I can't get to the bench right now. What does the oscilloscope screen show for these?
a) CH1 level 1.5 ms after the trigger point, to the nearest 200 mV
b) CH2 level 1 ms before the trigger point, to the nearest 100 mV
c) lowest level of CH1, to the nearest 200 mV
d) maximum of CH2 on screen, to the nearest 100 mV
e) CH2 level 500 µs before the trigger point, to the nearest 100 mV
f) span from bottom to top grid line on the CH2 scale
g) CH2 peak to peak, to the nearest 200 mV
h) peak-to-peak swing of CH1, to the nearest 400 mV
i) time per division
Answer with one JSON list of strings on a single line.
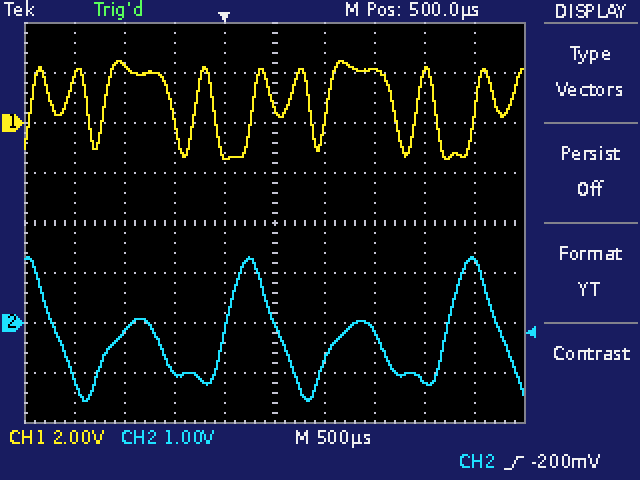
["2.2 V", "-200 mV", "-1.4 V", "1.3 V", "-1.0 V", "8 V", "2.8 V", "4.0 V", "500 µs"]
